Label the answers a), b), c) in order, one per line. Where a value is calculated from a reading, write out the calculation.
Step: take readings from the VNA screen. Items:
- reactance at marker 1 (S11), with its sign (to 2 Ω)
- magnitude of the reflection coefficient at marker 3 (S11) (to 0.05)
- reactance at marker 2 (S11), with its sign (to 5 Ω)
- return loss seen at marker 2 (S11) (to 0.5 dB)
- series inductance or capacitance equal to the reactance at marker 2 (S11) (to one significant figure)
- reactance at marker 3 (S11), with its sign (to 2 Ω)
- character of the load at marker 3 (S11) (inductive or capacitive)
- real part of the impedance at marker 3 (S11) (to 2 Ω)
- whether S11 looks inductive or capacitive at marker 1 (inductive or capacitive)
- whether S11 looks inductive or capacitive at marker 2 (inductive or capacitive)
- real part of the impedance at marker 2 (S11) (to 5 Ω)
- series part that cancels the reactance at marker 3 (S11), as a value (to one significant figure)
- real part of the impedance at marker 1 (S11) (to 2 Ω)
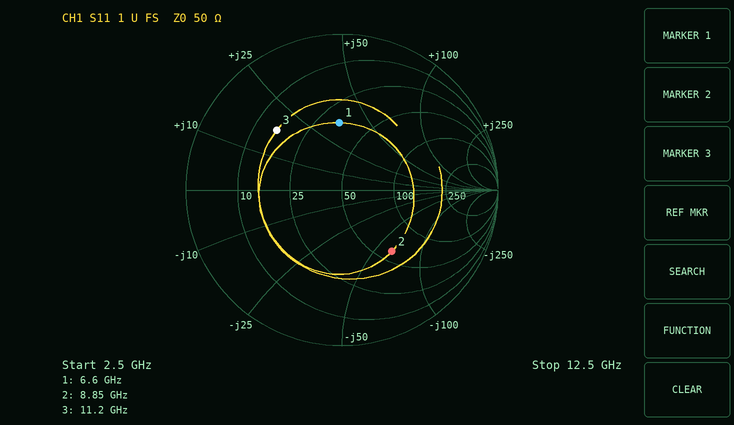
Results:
a) +36 Ω
b) 0.55
c) -65 Ω
d) 6.0 dB
e) C = 1/(2π × 8.85 GHz × 65 Ω) ≈ 277 fF, so 300 fF to one significant figure
f) +18 Ω
g) inductive
h) 16 Ω
i) inductive
j) capacitive
k) 60 Ω
l) C = 1/(2π × 11.2 GHz × 18 Ω) ≈ 789 fF, so 800 fF to one significant figure
m) 34 Ω
